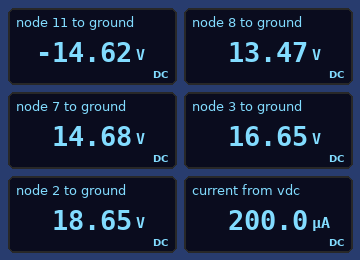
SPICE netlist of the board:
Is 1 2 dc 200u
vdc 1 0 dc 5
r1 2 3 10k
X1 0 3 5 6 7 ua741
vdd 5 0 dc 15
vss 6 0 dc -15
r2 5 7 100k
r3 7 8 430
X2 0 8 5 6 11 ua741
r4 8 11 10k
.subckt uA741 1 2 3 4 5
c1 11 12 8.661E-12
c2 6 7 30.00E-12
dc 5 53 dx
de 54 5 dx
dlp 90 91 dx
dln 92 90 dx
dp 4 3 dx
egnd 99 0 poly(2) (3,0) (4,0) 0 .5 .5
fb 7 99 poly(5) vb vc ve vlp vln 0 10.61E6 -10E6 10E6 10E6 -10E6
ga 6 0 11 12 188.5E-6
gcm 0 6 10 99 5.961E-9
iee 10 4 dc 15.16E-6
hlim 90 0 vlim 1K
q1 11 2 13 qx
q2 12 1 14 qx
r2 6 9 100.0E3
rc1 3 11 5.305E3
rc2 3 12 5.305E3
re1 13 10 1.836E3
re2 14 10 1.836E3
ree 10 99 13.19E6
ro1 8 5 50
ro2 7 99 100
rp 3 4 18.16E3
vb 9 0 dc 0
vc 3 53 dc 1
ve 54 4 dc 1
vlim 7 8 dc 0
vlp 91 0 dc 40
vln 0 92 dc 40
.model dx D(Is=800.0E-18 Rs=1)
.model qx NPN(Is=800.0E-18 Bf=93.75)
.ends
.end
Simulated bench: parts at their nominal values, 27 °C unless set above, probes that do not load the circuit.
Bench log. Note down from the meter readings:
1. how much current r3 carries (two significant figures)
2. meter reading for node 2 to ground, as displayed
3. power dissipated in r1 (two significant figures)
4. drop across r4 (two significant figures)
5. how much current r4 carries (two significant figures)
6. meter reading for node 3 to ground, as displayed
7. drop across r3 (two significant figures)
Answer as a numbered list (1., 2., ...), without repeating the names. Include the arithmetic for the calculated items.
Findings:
1. (14.68 V - 13.47 V) / 430 Ω = 2.8 mA
2. 18.65 V
3. (18.65 V - 16.65 V)^2 / 10 kΩ = 400 µW
4. 13.47 V - (-14.62 V) = 28 V
5. (13.47 V - (-14.62 V)) / 10 kΩ = 2.8 mA
6. 16.65 V
7. 14.68 V - 13.47 V = 1.2 V
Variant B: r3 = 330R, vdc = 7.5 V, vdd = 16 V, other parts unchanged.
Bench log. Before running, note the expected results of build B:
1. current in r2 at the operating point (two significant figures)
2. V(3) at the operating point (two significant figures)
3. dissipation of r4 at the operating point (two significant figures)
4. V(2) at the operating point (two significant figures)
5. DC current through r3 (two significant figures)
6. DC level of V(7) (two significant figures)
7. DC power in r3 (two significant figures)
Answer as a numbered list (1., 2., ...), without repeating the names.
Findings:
1. 3.2 µA
2. 18 V
3. 86 mW
4. 20 V
5. 2.9 mA
6. 16 V
7. 2.8 mW
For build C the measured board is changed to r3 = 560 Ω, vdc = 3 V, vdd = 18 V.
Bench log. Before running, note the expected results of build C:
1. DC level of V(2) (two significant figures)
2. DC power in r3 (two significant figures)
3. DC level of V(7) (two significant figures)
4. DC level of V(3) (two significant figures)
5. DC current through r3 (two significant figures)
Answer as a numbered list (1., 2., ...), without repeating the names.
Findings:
1. 22 V
2. 5.2 mW
3. 18 V
4. 20 V
5. 3.1 mA
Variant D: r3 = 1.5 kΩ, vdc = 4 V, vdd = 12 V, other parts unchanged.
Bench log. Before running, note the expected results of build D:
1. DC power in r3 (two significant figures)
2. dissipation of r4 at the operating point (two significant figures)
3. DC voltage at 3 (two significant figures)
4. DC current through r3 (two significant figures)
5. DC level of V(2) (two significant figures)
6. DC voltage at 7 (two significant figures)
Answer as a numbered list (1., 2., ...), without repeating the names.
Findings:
1. 7.8 mW
2. 52 mW
3. 14 V
4. 2.3 mA
5. 16 V
6. 12 V
